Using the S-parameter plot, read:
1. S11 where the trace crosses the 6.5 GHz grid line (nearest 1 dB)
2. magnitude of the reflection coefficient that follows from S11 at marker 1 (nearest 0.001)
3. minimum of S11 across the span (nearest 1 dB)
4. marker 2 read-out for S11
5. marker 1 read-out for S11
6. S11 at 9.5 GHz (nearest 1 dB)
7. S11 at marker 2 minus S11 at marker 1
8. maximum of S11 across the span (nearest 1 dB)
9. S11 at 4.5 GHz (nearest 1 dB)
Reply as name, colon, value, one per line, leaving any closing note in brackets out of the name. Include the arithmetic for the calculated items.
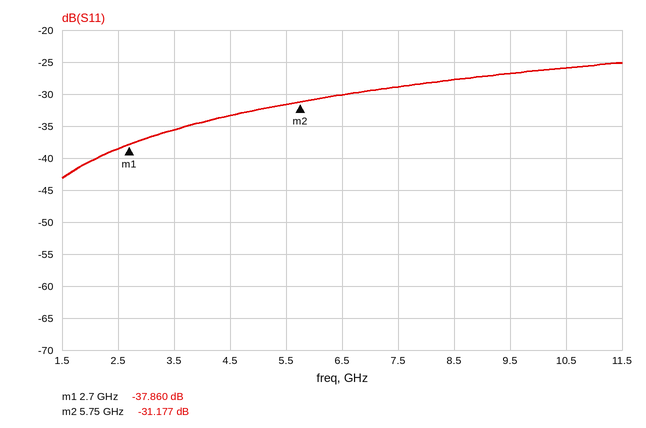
S11 where the trace crosses the 6.5 GHz grid line: -30 dB
magnitude of the reflection coefficient that follows from S11 at marker 1: 10^(-37.86/20) ≈ 0.013
minimum of S11 across the span: -43 dB
marker 2 read-out for S11: -31.177 dB
marker 1 read-out for S11: -37.860 dB
S11 at 9.5 GHz: -27 dB
S11 at marker 2 minus S11 at marker 1: -31.177 − (-37.86) = 6.683 dB
maximum of S11 across the span: -25 dB
S11 at 4.5 GHz: -33 dB
